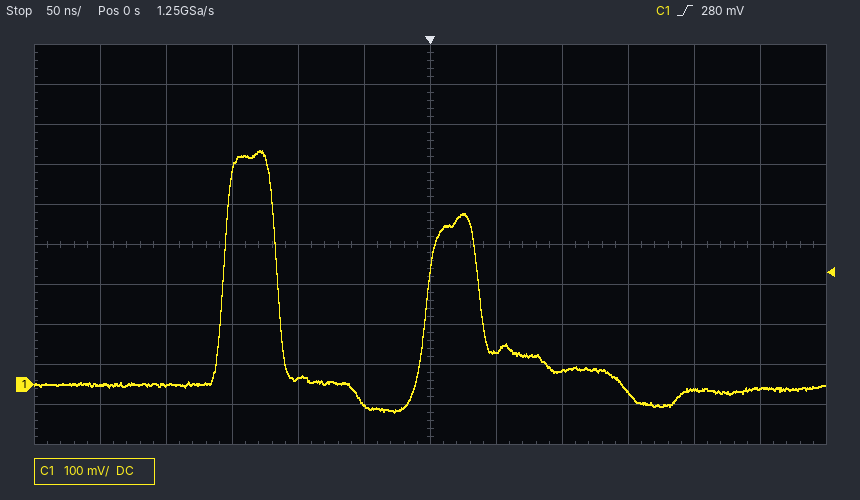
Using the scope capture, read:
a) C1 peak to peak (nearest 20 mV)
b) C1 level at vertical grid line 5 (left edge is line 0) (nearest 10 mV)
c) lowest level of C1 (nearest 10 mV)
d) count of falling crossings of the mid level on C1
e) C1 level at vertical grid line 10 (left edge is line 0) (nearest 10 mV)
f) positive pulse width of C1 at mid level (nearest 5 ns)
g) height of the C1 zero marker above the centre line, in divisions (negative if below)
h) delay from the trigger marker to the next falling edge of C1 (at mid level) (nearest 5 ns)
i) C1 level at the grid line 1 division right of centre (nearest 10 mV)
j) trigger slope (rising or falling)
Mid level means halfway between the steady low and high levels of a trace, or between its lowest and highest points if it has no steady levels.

660 mV
-50 mV
-70 mV
2
-10 mV
40 ns
-3.5 div
35 ns
80 mV
rising
